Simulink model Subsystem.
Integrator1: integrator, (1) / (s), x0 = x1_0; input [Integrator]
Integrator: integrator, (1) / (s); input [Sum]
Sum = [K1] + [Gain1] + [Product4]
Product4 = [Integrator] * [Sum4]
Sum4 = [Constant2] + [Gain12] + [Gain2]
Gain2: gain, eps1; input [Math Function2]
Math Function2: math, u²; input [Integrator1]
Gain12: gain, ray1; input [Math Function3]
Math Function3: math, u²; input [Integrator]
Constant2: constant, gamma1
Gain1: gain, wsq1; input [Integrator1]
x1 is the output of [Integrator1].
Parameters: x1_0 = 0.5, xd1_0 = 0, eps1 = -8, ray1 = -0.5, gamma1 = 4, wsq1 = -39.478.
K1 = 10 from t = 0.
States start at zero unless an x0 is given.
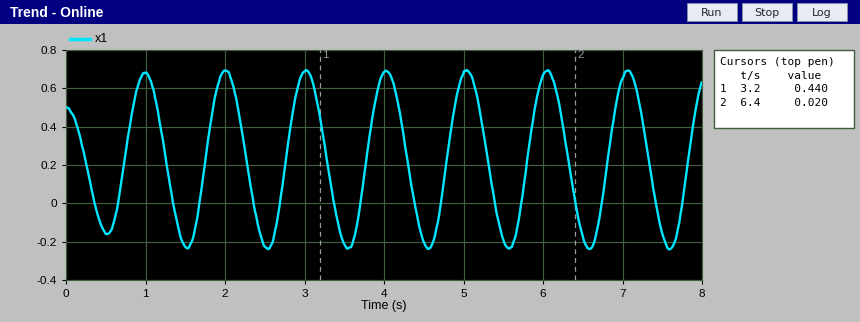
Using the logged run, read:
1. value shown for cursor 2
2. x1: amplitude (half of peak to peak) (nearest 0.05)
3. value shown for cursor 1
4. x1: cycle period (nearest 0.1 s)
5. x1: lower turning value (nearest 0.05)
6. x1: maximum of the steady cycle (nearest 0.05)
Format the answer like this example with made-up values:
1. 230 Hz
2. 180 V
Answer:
1. 0.020
2. 0.45
3. 0.440
4. 1.0 s
5. -0.25
6. 0.70
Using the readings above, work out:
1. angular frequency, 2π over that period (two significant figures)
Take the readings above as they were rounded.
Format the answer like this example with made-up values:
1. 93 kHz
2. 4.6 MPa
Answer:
1. 6.3 rad/s
